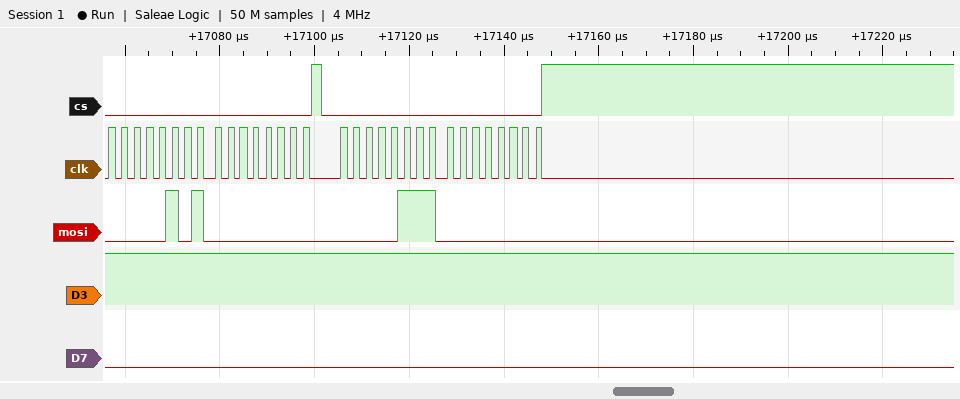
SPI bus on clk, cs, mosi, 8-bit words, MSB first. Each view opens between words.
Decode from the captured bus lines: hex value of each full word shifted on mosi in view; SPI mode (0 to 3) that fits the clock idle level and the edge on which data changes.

05, 00, 07, 00
0
